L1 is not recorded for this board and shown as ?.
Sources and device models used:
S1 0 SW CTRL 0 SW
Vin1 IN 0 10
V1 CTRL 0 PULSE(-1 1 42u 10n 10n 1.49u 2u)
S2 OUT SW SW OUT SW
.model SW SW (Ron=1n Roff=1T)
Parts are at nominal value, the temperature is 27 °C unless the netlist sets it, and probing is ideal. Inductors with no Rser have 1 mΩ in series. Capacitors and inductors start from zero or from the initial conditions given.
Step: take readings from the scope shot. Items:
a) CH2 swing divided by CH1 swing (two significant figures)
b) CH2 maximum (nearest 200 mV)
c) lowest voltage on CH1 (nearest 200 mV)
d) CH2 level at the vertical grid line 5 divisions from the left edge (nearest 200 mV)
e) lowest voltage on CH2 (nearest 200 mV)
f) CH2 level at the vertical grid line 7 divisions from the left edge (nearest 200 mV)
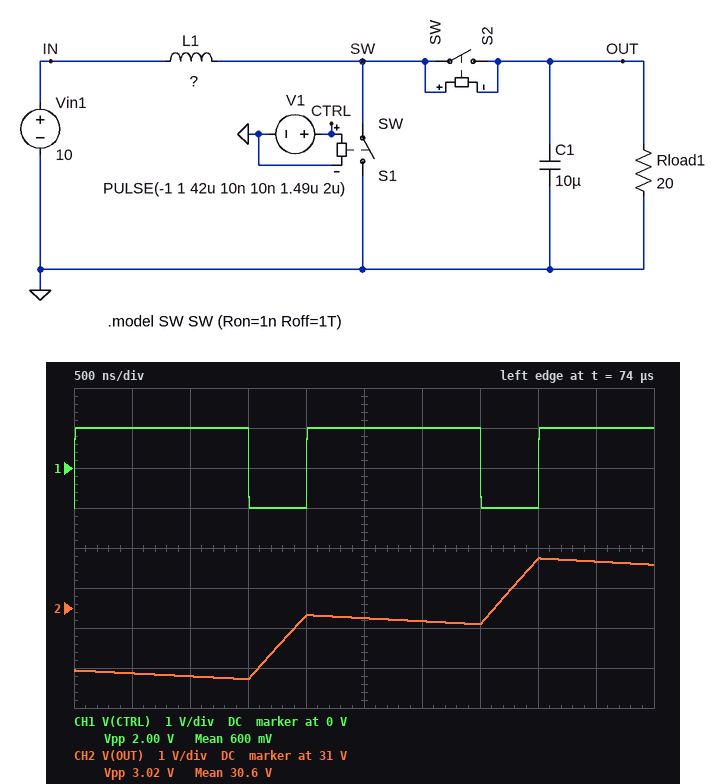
1.5
32.2 V
-1.0 V
30.8 V
29.2 V
30.6 V
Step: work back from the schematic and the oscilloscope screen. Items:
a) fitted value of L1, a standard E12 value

4.7 µH
